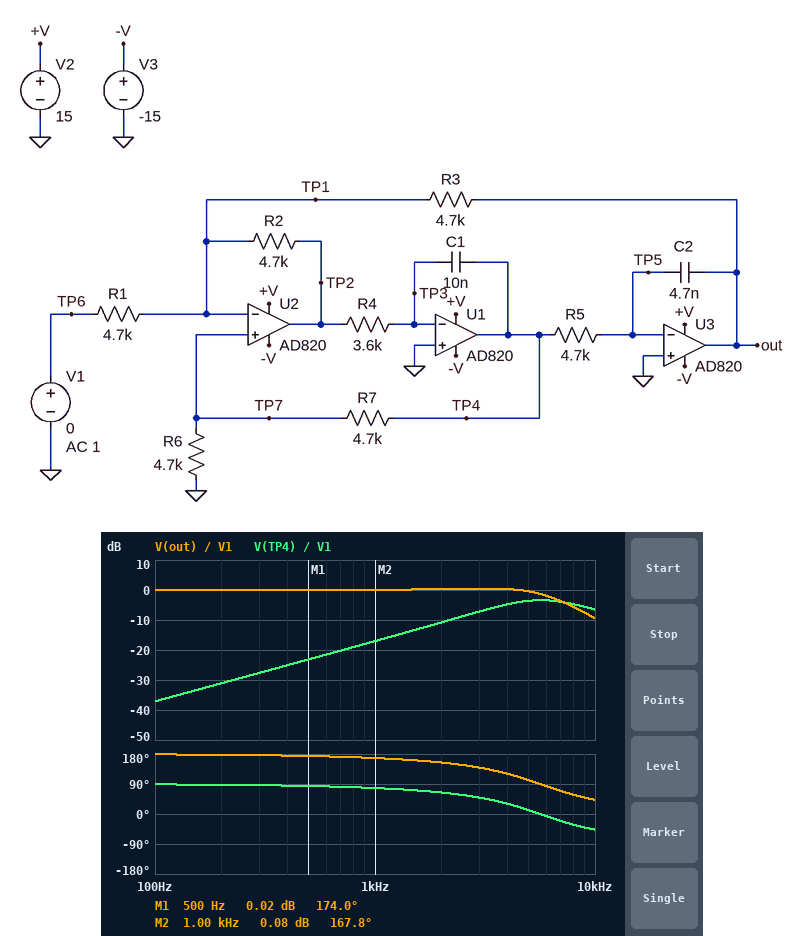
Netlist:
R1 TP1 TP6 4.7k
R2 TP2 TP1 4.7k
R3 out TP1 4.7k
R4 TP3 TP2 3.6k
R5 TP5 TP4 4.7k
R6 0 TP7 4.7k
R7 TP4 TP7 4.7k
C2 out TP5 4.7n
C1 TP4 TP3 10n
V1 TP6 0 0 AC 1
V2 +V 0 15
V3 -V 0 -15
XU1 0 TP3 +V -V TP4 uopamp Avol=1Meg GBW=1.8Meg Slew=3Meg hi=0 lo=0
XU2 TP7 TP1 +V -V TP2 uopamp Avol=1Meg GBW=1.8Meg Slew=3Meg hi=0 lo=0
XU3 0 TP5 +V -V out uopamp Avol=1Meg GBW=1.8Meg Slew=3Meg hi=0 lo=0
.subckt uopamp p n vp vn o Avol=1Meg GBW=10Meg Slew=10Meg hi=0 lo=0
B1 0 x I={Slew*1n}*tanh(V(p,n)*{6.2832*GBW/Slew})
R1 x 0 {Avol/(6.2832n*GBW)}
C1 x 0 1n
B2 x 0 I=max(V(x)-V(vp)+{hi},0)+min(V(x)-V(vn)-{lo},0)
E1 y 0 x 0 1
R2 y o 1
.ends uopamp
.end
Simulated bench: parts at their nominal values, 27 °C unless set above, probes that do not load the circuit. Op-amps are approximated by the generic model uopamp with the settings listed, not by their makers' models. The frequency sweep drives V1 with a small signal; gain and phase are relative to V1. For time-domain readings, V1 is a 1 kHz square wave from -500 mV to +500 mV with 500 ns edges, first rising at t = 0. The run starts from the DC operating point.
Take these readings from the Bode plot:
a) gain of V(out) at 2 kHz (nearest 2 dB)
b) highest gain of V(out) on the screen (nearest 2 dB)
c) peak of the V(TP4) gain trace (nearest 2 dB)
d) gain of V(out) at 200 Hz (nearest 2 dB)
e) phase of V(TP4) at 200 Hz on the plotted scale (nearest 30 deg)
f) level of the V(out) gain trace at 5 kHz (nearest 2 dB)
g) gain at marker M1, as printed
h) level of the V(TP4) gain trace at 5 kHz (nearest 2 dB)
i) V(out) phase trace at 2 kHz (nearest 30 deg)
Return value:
0 dB
0 dB
-4 dB
0 dB
90 deg
0 dB
0.02 dB
-4 dB
150 deg
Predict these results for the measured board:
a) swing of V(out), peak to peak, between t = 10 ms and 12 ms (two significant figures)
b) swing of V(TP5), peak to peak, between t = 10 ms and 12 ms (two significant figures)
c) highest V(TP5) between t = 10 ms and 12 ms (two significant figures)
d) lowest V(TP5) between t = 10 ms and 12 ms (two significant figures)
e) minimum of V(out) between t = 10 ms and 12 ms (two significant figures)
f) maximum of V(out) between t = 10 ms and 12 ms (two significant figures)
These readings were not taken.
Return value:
1.2 V
3.2 mV
1.6 mV
-1.6 mV
-600 mV
600 mV
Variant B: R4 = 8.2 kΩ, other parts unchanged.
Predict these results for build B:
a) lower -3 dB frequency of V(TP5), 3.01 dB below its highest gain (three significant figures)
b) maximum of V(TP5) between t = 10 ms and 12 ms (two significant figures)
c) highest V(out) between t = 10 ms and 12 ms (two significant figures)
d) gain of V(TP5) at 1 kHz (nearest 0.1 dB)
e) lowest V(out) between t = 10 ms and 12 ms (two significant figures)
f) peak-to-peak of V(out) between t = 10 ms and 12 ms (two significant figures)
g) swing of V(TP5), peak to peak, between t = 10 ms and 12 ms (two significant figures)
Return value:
2.57 kHz
1.3 mV
770 mV
-64.7 dB
-770 mV
1.5 V
2.6 mV
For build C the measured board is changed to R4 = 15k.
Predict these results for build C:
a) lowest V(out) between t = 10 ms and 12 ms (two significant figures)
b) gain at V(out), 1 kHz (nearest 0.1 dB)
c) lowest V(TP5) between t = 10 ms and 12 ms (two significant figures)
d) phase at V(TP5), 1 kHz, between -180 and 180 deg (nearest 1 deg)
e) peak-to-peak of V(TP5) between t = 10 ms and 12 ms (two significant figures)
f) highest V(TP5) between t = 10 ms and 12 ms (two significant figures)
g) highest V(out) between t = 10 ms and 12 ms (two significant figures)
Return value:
-900 mV
1.0 dB
-1.1 mV
76 deg
2.1 mV
1.1 mV
900 mV
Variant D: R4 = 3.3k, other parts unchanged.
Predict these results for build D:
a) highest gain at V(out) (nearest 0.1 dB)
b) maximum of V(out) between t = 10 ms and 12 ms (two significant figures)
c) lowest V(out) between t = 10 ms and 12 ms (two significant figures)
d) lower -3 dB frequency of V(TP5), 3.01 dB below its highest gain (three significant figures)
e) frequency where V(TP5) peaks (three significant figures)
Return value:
0.3 dB
590 mV
-590 mV
3.32 kHz
5.92 kHz
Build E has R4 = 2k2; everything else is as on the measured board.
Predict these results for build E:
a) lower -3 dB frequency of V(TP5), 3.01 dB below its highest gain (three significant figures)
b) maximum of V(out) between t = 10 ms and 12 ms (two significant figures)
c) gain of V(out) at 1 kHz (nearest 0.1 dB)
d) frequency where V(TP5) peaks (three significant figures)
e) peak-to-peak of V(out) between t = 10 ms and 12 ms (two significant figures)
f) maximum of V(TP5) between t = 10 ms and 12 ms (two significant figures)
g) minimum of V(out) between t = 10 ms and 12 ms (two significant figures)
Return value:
3.64 kHz
530 mV
0 dB
7.28 kHz
1.1 V
1.8 mV
-530 mV
